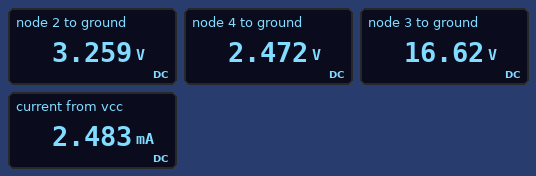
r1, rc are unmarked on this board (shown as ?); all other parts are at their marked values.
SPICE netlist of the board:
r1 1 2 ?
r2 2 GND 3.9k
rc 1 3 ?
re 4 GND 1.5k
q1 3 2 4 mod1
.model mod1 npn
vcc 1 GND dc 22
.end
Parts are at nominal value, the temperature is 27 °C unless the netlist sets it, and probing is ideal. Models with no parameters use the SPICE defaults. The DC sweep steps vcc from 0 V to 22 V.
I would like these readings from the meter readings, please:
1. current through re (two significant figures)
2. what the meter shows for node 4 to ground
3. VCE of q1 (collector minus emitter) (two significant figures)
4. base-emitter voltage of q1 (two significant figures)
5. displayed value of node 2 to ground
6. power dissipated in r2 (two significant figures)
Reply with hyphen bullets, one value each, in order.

- 1.6 mA
- 2.472 V
- 14 V
- 790 mV
- 3.259 V
- 2.7 mW
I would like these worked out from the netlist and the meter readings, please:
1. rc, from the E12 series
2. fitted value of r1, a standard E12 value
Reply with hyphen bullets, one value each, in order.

- 3.3 kΩ
- 22 kΩ
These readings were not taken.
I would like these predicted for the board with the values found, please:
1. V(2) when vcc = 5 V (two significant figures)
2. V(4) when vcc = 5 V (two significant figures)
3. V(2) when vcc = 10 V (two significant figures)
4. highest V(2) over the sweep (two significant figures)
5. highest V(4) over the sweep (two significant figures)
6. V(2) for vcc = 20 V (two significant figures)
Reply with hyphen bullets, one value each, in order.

- 750 mV
- 61 mV
- 1.5 V
- 3.3 V
- 2.5 V
- 3.0 V
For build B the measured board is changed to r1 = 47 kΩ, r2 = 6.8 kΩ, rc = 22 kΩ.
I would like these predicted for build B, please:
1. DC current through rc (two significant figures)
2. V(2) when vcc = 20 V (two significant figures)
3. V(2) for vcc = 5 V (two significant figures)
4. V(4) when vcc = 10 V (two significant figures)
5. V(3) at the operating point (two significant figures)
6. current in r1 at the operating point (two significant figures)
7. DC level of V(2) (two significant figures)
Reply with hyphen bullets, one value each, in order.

- 930 µA
- 2.1 V
- 630 mV
- 500 mV
- 1.6 V
- 420 µA
- 2.3 V
